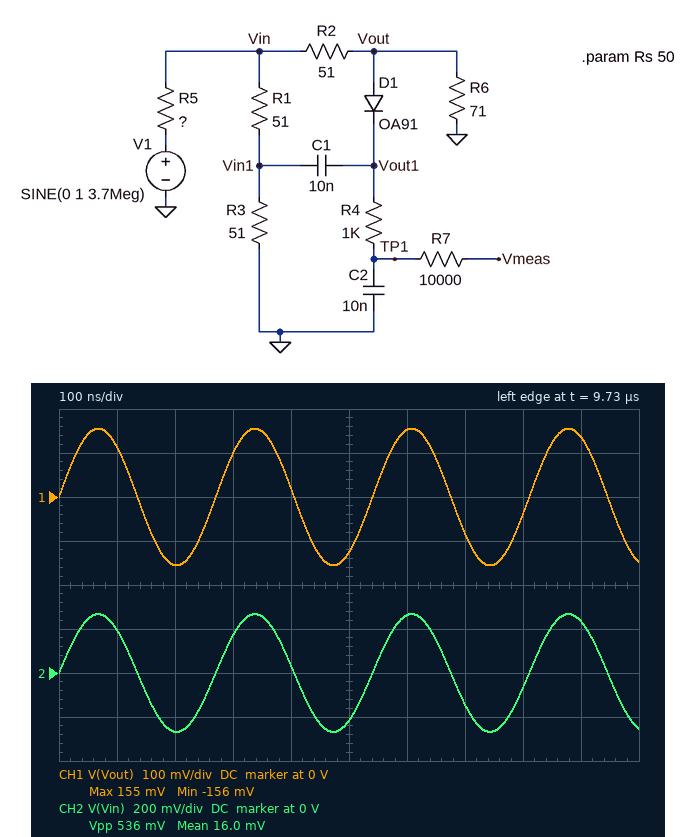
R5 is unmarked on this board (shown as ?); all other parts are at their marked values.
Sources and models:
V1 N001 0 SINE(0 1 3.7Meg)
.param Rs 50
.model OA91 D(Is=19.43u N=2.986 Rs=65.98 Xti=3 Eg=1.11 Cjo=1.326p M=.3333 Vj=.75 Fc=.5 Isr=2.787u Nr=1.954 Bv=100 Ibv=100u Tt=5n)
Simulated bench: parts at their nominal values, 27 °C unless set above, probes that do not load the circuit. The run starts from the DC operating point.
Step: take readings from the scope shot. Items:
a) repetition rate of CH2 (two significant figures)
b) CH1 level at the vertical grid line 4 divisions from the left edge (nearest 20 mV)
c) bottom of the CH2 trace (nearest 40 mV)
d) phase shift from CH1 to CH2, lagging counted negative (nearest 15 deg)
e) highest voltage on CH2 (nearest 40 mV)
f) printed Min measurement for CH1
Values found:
3.7 MHz
20 mV
-280 mV
0 deg
280 mV
-156 mV
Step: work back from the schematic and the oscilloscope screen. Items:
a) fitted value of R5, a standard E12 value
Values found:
150 Ω
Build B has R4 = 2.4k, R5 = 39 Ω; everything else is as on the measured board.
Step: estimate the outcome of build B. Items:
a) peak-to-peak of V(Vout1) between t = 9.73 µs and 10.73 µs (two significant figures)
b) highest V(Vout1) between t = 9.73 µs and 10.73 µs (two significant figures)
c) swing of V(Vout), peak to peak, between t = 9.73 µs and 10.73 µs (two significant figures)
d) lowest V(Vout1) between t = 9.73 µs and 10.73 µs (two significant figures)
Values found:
580 mV
290 mV
680 mV
-290 mV
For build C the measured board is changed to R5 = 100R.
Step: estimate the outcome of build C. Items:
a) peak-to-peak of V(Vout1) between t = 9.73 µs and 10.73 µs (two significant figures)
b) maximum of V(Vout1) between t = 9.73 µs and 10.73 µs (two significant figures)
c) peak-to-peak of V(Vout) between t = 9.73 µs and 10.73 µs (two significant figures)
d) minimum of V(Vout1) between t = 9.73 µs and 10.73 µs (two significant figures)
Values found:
350 mV
170 mV
410 mV
-170 mV
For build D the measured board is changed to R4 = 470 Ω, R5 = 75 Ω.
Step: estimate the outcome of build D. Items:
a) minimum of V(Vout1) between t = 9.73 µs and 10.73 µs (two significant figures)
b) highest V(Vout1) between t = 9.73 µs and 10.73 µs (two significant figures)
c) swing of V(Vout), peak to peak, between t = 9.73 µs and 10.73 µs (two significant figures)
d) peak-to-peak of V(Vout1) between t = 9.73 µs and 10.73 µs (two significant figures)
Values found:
-200 mV
200 mV
490 mV
400 mV
